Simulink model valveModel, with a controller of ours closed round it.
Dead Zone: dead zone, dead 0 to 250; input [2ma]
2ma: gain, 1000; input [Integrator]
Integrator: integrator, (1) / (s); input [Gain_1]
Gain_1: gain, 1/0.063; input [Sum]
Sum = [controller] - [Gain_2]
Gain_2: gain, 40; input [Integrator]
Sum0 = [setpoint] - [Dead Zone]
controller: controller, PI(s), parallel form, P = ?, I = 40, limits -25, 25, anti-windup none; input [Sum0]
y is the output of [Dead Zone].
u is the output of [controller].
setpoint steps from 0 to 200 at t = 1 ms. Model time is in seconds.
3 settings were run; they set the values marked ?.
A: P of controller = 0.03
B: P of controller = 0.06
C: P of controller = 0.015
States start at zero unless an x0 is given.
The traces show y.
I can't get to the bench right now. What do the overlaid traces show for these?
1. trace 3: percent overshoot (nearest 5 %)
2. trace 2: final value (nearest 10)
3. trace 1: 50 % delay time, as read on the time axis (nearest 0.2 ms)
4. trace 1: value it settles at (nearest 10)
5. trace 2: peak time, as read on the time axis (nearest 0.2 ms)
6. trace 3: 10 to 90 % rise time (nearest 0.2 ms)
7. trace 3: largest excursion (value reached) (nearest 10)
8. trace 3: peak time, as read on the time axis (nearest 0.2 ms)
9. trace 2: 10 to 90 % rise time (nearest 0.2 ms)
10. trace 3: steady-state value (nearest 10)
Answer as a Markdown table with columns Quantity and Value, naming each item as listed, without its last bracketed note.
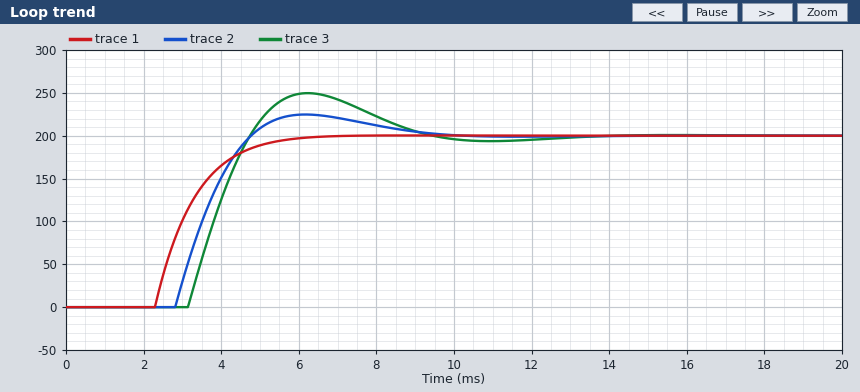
| Quantity | Value |
|---|---|
| trace 3: percent overshoot | 25 % |
| trace 2: final value | 200 |
| trace 1: 50 % delay time, as read on the time axis | 3.0 ms |
| trace 1: value it settles at | 200 |
| trace 2: peak time, as read on the time axis | 6.2 ms |
| trace 3: 10 to 90 % rise time | 1.2 ms |
| trace 3: largest excursion (value reached) | 250 |
| trace 3: peak time, as read on the time axis | 6.2 ms |
| trace 2: 10 to 90 % rise time | 1.4 ms |
| trace 3: steady-state value | 200 |
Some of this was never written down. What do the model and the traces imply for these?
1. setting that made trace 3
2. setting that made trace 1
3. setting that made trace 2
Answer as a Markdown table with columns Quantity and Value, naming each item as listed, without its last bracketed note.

| Quantity | Value |
|---|---|
| setting that made trace 3 | C |
| setting that made trace 1 | B |
| setting that made trace 2 | A |
